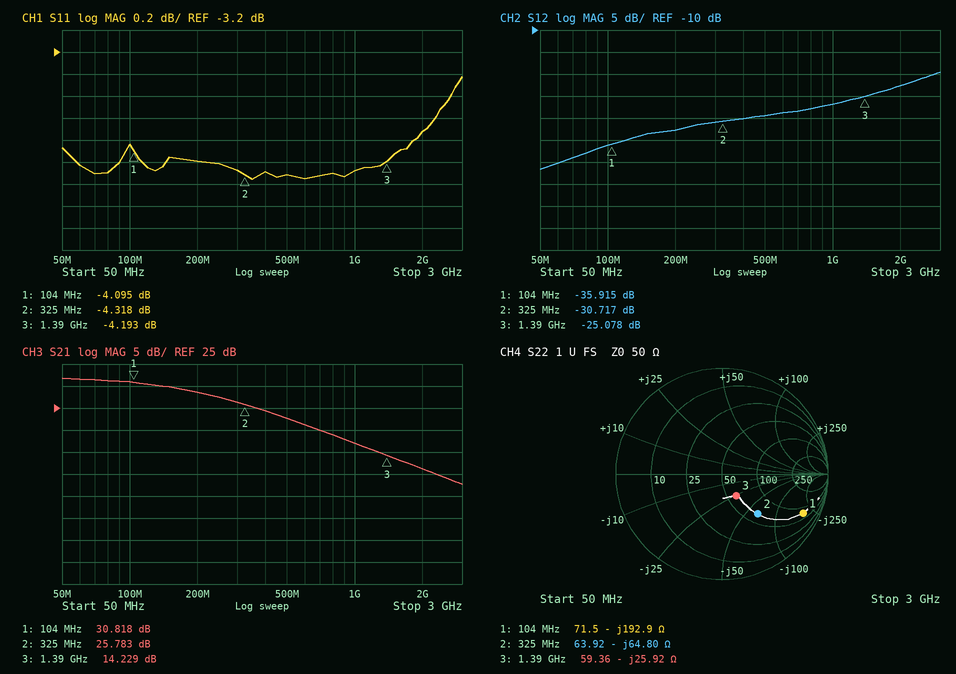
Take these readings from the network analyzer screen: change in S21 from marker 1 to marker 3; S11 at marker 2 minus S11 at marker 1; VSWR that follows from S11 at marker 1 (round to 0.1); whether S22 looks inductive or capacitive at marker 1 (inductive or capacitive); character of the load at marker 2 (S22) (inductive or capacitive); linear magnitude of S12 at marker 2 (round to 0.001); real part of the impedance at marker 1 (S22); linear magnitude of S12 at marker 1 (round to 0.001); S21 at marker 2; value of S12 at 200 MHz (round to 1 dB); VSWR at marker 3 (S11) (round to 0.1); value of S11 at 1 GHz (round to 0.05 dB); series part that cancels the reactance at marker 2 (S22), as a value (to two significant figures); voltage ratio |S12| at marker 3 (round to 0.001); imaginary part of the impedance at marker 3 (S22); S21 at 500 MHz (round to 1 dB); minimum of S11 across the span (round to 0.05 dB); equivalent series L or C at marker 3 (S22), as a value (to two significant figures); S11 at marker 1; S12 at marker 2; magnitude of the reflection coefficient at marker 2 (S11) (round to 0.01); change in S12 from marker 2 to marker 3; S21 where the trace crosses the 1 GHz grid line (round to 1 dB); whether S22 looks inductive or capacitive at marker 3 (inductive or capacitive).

-16.589 dB
-0.223 dB
4.3
capacitive
capacitive
0.029
71.5 Ω
0.016
25.783 dB
-33 dB
4.2
-4.30 dB
32 nH
0.056
-25.92 Ω
23 dB
-4.35 dB
4.4 pF
-4.095 dB
-30.717 dB
0.61
5.639 dB
17 dB
capacitive
